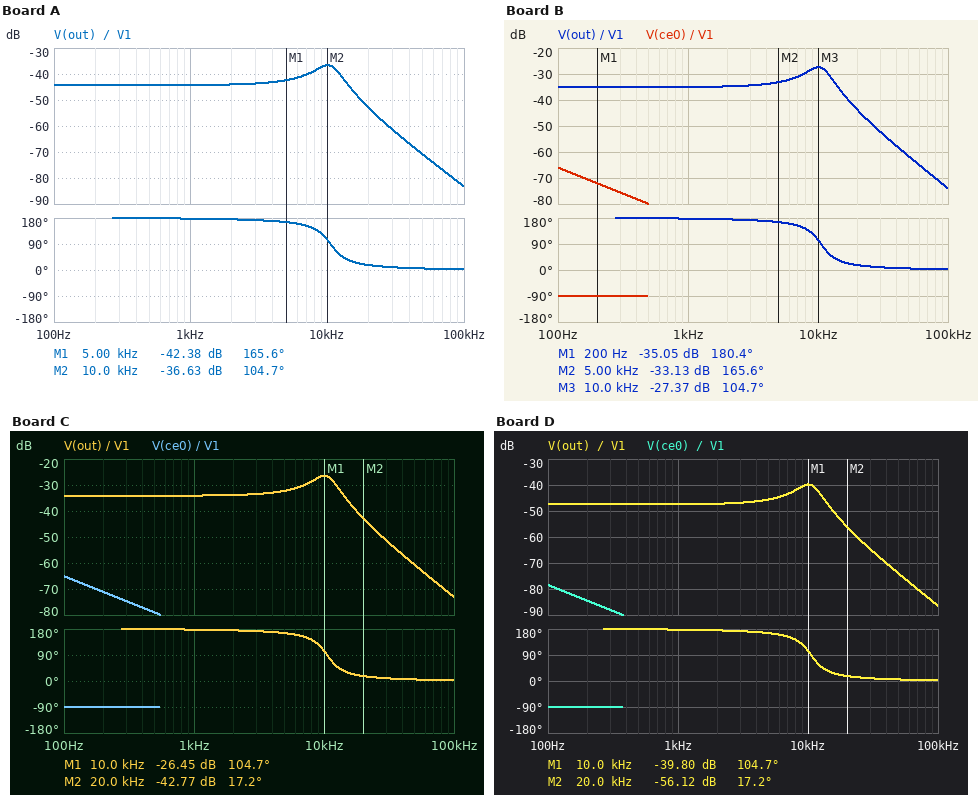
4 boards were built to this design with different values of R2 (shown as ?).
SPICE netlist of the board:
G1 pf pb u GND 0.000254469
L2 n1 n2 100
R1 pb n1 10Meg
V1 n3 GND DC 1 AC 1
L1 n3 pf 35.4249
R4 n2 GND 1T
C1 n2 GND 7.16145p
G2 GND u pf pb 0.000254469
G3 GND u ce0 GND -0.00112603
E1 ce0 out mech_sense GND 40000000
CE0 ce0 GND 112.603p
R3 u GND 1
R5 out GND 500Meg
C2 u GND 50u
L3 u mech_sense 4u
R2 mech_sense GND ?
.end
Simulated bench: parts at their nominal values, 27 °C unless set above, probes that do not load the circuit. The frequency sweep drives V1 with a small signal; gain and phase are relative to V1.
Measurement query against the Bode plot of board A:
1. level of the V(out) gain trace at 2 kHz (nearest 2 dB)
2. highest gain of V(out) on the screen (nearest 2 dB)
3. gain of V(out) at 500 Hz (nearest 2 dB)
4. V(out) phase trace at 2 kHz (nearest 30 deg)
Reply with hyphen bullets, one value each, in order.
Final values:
- -44 dB
- -36 dB
- -44 dB
- 180 deg
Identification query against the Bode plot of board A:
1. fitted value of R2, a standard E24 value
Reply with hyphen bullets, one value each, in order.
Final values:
- 620 nΩ
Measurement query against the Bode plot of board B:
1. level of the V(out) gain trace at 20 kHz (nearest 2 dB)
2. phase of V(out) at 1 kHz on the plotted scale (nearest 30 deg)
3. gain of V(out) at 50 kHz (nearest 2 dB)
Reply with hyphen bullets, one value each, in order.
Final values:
- -44 dB
- 180 deg
- -62 dB
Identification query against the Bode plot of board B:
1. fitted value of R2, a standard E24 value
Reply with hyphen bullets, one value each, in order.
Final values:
- 1.8 µΩ
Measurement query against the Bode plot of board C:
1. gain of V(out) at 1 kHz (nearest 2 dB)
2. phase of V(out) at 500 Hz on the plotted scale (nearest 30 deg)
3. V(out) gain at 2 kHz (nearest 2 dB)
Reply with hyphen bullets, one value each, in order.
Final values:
- -34 dB
- 180 deg
- -34 dB
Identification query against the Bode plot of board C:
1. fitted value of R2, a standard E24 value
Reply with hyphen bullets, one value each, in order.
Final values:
- 2 µΩ
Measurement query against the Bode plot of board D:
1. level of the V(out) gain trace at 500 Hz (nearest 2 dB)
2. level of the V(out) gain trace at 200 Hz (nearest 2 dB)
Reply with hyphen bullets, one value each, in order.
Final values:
- -48 dB
- -48 dB
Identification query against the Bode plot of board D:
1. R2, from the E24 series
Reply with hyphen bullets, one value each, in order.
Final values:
- 430 nΩ
